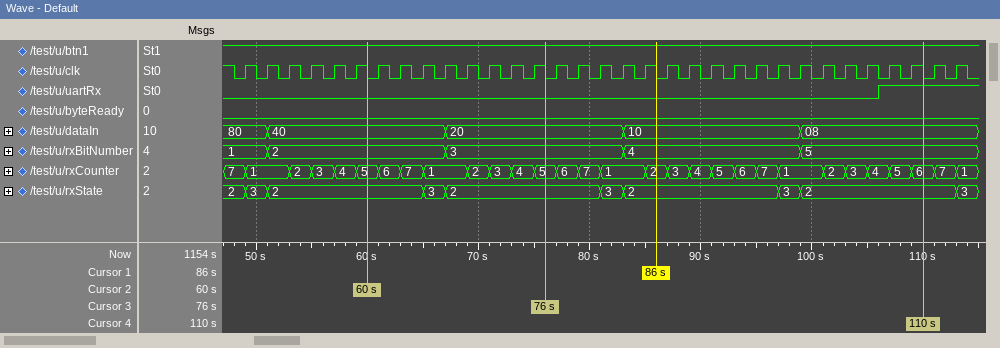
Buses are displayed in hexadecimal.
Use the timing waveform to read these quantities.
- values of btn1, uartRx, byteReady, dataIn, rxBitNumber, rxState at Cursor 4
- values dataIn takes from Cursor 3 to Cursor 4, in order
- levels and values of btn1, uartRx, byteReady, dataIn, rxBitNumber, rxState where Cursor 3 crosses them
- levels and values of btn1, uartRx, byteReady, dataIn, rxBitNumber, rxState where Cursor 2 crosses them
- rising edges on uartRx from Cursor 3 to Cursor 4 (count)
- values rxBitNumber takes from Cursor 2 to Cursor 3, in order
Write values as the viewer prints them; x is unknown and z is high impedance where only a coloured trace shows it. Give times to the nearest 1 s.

btn1=1, uartRx=1, byteReady=0, dataIn=08, rxBitNumber=5, rxState=2
20, 10, 08
btn1=1, uartRx=0, byteReady=0, dataIn=20, rxBitNumber=3, rxState=2
btn1=1, uartRx=0, byteReady=0, dataIn=40, rxBitNumber=2, rxState=2
1
2, 3
